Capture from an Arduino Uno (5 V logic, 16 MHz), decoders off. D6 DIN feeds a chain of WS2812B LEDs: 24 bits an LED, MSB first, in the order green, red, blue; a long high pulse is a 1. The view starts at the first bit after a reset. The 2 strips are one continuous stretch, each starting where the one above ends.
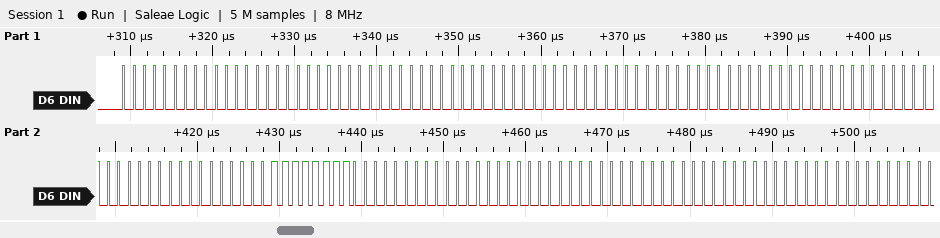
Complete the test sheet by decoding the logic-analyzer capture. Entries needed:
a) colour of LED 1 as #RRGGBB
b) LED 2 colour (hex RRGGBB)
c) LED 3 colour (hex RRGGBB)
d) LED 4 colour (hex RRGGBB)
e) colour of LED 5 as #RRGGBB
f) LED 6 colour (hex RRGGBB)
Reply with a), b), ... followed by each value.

a) #000000
b) #000000
c) #000000
d) #000000
e) #00FF00
f) #000000
